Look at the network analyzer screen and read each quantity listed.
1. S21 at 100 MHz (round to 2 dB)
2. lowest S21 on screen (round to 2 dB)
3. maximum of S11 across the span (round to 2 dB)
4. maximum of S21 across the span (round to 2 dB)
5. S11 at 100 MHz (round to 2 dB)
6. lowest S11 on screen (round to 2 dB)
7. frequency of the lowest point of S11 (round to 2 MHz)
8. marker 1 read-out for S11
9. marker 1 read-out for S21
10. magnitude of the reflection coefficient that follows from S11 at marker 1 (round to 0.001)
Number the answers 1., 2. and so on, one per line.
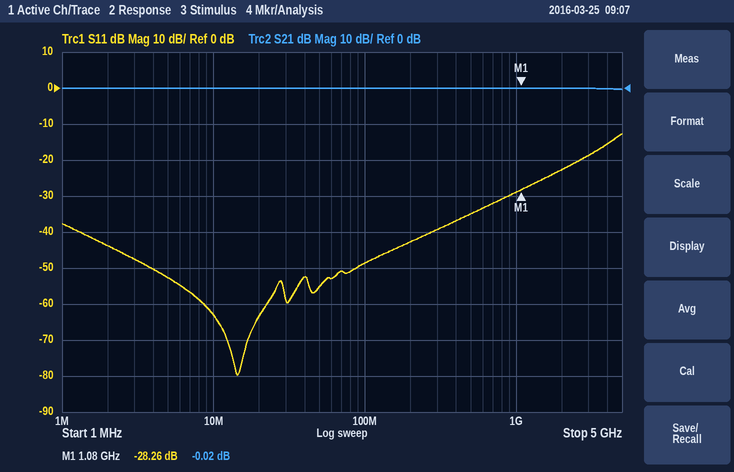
1. 0 dB
2. 0 dB
3. -12 dB
4. 0 dB
5. -48 dB
6. -80 dB
7. 14 MHz
8. -28.26 dB
9. -0.02 dB
10. 0.039
